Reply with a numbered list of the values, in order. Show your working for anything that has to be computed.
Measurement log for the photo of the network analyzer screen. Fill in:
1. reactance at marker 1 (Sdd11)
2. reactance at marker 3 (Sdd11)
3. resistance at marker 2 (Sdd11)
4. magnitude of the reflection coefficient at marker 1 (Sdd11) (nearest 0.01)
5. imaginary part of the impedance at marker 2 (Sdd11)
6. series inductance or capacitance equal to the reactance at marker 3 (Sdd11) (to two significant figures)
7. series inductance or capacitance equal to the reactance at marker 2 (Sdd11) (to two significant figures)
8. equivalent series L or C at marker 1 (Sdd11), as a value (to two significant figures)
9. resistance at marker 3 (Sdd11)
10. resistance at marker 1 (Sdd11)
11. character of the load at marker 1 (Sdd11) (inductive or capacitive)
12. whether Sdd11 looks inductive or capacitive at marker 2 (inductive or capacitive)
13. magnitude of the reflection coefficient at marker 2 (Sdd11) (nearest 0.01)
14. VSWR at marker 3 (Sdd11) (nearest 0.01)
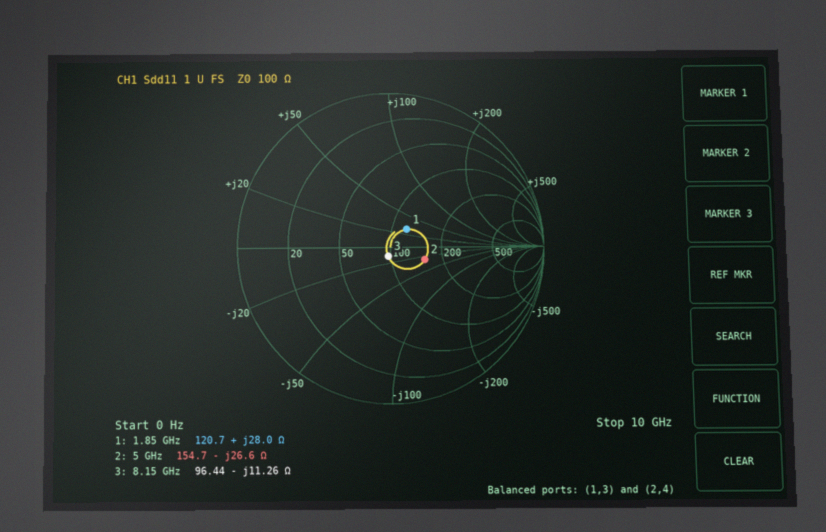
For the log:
1. +28.0 Ω
2. -11.26 Ω
3. 154.7 Ω
4. 0.16
5. -26.6 Ω
6. C = 1/(2π × 8.15 GHz × 11.26 Ω) ≈ 1.7 pF
7. C = 1/(2π × 5 GHz × 26.6 Ω) ≈ 1.2 pF
8. L = 28 Ω/(2π × 1.85 GHz) ≈ 2.4 nH
9. 96.44 Ω
10. 120.7 Ω
11. inductive
12. capacitive
13. 0.24
14. 1.13
